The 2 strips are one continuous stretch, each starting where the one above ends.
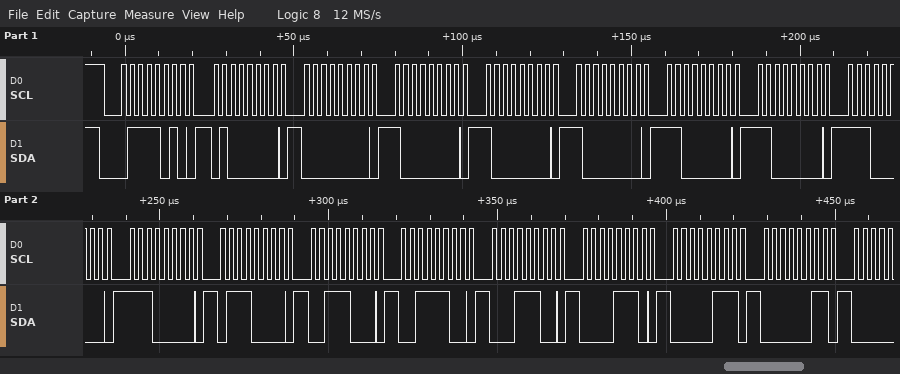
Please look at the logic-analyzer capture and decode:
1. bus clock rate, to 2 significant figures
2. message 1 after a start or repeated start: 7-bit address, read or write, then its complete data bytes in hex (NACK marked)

400 kHz
0x3D write: 40 00 80 80 80 C0 C0 E0 E0 70 38 3C 1C 0E 07 03
